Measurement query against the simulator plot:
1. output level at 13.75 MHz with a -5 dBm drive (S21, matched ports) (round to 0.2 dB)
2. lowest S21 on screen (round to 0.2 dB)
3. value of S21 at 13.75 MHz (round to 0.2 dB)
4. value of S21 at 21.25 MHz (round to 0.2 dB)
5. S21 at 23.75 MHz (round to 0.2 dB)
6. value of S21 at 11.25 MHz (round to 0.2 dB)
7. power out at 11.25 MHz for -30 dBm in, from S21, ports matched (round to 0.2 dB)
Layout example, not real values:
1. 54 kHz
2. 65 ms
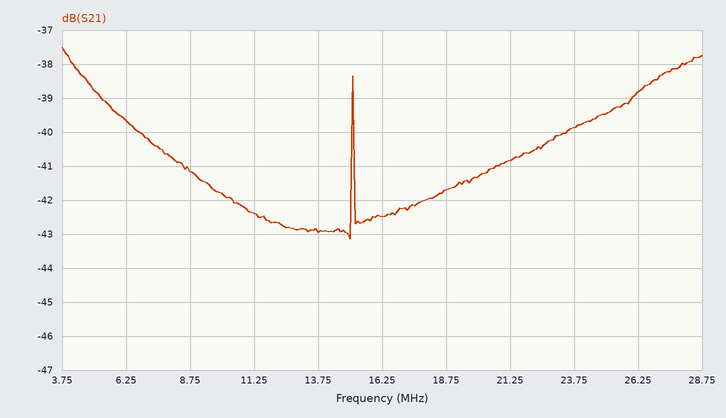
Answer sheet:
1. -48.0 dBm
2. -43.2 dB
3. -43.0 dB
4. -40.8 dB
5. -39.8 dB
6. -42.4 dB
7. -72.4 dBm
